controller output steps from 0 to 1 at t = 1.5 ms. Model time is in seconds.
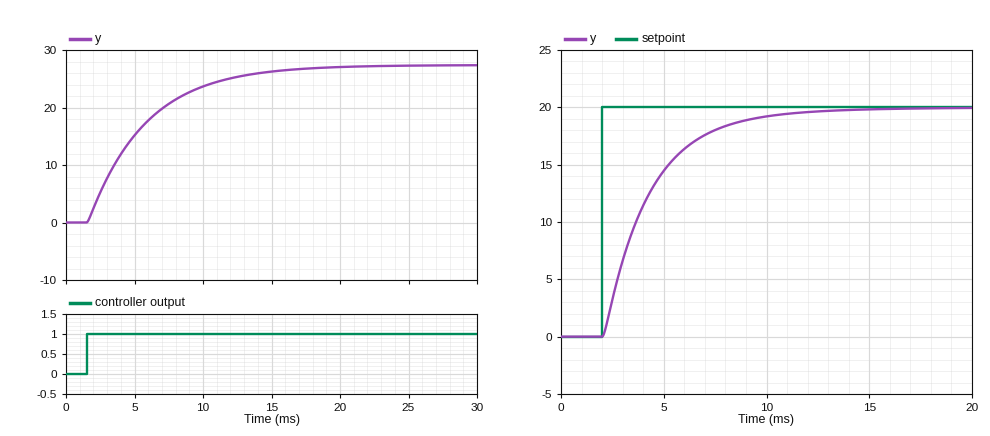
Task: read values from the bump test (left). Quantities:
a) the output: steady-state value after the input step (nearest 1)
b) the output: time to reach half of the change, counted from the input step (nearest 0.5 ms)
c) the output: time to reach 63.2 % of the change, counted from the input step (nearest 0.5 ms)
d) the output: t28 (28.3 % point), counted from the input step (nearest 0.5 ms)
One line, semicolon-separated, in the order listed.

27; 3.0 ms; 4.5 ms; 1.5 ms
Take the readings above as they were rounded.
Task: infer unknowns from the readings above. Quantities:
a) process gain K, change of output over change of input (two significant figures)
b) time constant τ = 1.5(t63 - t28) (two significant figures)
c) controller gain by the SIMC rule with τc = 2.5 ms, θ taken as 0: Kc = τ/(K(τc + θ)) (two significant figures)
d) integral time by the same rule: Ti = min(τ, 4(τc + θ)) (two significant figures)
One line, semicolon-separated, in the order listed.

27; 4.5 ms; 0.067; 4.5 ms
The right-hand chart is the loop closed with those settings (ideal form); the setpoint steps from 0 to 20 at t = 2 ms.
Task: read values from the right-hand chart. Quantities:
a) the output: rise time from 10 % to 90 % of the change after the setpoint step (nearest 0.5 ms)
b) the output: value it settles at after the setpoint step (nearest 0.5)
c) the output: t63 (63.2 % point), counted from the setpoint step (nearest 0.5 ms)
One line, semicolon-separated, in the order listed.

5.0 ms; 20.0; 2.5 ms
